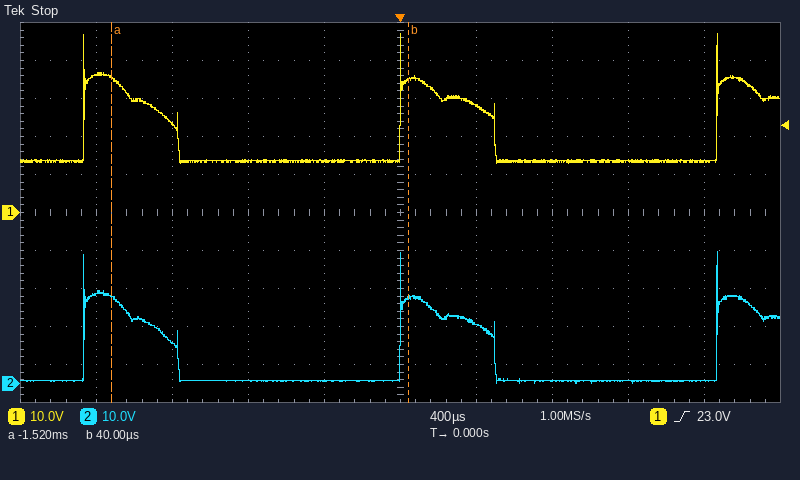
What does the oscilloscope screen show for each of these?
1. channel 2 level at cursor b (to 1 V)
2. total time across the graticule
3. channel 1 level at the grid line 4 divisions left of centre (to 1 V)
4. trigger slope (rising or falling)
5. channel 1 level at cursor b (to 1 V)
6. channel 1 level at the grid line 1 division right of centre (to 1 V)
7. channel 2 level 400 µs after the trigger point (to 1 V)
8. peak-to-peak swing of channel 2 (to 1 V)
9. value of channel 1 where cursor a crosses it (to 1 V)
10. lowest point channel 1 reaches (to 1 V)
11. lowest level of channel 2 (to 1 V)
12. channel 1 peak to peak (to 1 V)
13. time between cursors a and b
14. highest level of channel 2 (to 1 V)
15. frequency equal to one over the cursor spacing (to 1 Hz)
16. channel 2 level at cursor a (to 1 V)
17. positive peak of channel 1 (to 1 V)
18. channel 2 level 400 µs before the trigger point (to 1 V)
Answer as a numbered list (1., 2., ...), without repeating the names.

1. 22 V
2. 4 ms
3. 36 V
4. rising
5. 35 V
6. 28 V
7. 16 V
8. 35 V
9. 35 V
10. 13 V
11. 0 V
12. 34 V
13. 1.56 ms
14. 35 V
15. 641 Hz
16. 23 V
17. 47 V
18. 1 V
